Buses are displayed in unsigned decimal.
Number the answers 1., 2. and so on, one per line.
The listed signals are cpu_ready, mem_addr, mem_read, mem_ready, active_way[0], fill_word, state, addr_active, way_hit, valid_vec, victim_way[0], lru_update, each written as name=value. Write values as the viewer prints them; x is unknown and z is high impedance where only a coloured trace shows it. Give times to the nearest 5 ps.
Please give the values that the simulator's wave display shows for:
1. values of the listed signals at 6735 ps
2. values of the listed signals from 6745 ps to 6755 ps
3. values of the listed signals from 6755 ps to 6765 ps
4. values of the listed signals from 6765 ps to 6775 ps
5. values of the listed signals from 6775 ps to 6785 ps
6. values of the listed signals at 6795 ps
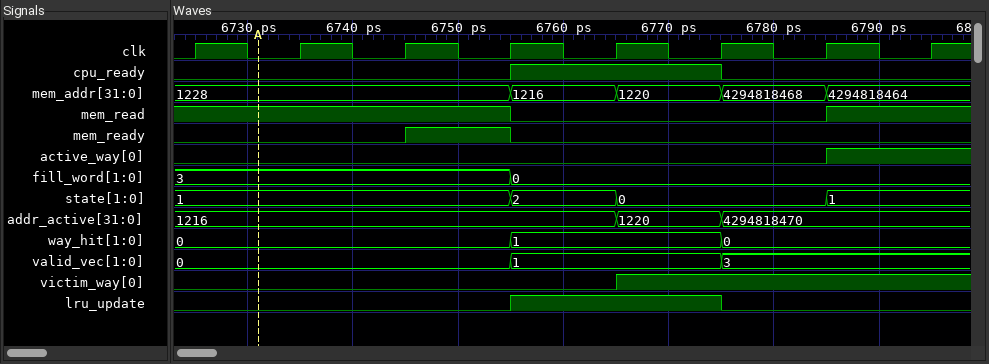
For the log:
1. cpu_ready=0, mem_addr=1228, mem_read=1, mem_ready=0, active_way[0]=0, fill_word=3, state=1, addr_active=1216, way_hit=0, valid_vec=0, victim_way[0]=0, lru_update=0
2. cpu_ready=0, mem_addr=1228, mem_read=1, mem_ready=1, active_way[0]=0, fill_word=3, state=1, addr_active=1216, way_hit=0, valid_vec=0, victim_way[0]=0, lru_update=0
3. cpu_ready=1, mem_addr=1216, mem_read=0, mem_ready=0, active_way[0]=0, fill_word=0, state=2, addr_active=1216, way_hit=1, valid_vec=1, victim_way[0]=0, lru_update=1
4. cpu_ready=1, mem_addr=1220, mem_read=0, mem_ready=0, active_way[0]=0, fill_word=0, state=0, addr_active=1220, way_hit=1, valid_vec=1, victim_way[0]=1, lru_update=1
5. cpu_ready=0, mem_addr=4294818468, mem_read=0, mem_ready=0, active_way[0]=0, fill_word=0, state=0, addr_active=4294818470, way_hit=0, valid_vec=3, victim_way[0]=1, lru_update=0
6. cpu_ready=0, mem_addr=4294818464, mem_read=1, mem_ready=0, active_way[0]=1, fill_word=0, state=1, addr_active=4294818470, way_hit=0, valid_vec=3, victim_way[0]=1, lru_update=0
